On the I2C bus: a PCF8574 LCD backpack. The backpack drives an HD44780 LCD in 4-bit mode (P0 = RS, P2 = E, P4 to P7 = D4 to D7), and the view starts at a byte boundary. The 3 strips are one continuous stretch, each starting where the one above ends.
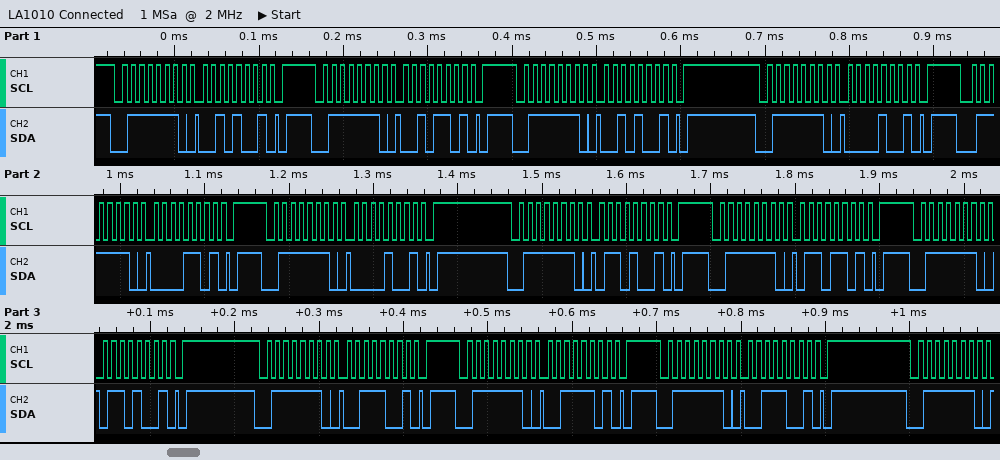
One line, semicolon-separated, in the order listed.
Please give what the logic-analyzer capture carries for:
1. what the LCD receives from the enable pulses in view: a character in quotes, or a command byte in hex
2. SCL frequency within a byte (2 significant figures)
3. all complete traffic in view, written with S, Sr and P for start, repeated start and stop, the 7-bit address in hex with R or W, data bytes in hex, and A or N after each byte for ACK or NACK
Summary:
' ' 'c'; 100 kHz; S 3FW A 29 A P S 3FW A 2D A P S 3FW A 29 A P S 3FW A 09 A P S 3FW A 0D A P S 3FW A 09 A P S 3FW A 69 A P S 3FW A 6D A P S 3FW A 69 A P S 3FW A 39 A P S 3FW A 3D A P S 3FW A 39 A P S 3FW A
